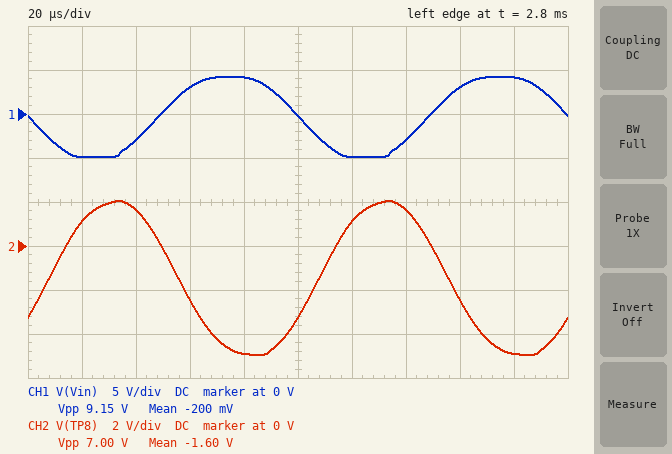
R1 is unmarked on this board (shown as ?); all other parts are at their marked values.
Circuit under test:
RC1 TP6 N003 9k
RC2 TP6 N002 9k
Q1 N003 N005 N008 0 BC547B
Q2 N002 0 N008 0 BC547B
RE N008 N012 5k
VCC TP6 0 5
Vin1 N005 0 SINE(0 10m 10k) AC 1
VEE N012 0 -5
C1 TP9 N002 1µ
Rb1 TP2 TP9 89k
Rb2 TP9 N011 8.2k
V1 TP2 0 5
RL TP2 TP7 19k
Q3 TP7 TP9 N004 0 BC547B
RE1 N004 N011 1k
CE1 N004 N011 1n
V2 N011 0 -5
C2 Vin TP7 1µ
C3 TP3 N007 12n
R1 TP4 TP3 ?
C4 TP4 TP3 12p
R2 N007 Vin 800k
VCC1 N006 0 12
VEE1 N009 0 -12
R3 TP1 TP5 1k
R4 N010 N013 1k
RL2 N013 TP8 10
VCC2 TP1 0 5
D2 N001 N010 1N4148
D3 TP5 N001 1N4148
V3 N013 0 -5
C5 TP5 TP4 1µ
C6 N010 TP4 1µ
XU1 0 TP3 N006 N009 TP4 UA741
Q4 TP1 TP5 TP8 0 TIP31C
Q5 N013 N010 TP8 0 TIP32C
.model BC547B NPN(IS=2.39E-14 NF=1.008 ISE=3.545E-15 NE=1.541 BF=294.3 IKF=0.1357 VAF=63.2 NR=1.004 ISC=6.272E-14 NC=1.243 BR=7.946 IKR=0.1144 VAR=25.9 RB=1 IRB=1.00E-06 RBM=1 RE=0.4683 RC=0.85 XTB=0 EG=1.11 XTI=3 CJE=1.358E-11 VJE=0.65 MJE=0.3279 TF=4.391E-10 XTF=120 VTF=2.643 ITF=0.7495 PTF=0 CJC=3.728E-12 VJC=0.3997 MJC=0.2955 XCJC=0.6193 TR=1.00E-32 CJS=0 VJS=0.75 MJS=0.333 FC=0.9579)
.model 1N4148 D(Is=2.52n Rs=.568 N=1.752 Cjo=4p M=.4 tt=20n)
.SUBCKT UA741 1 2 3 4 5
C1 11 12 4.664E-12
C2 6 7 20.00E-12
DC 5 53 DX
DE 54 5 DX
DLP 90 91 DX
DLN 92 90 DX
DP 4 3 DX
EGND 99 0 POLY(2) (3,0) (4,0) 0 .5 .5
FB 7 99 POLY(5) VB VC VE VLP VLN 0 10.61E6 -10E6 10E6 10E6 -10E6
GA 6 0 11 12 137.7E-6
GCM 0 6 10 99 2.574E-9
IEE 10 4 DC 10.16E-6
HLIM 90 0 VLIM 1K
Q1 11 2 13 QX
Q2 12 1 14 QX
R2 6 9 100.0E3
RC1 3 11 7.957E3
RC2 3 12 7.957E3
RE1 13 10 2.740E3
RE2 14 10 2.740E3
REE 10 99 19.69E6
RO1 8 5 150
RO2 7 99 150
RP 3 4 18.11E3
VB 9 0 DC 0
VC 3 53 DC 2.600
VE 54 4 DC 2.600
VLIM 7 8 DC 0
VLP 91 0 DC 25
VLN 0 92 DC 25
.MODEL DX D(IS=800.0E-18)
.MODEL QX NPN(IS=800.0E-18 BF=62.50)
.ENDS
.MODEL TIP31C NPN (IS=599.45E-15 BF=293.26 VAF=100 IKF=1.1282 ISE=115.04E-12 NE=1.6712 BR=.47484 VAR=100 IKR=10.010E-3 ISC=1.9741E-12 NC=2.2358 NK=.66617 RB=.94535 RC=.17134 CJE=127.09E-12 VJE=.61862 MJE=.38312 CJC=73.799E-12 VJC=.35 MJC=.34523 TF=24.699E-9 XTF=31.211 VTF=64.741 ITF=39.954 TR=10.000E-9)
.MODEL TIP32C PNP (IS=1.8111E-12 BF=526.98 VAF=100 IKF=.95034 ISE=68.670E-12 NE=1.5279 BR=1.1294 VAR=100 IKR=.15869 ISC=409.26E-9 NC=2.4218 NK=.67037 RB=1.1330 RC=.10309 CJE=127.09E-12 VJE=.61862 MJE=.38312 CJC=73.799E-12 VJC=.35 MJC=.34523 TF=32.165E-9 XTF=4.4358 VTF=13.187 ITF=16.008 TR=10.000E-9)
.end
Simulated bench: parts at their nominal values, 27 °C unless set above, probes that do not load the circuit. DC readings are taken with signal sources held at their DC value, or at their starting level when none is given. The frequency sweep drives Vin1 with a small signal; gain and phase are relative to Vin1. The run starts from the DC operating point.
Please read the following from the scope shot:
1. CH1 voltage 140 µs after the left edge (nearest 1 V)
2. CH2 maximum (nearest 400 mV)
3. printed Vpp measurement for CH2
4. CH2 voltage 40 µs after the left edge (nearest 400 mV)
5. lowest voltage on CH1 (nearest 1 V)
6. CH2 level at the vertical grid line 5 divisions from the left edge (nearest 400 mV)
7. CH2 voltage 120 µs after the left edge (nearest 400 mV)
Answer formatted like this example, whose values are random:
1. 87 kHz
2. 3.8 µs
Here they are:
1. -3 V
2. 2.0 V
3. 7.00 V
4. 1.6 V
5. -5 V
6. -3.2 V
7. 1.2 V
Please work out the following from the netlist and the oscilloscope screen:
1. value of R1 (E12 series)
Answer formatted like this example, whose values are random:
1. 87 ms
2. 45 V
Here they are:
1. 680 kΩ
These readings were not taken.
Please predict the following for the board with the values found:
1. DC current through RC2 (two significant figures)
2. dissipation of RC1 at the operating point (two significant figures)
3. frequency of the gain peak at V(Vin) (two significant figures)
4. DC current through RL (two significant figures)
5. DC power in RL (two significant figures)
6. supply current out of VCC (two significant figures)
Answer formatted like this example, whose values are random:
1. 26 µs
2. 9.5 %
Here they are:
1. 440 µA
2. 1.7 mW
3. 420 kHz
4. 240 µA
5. 1.1 mW
6. 870 µA
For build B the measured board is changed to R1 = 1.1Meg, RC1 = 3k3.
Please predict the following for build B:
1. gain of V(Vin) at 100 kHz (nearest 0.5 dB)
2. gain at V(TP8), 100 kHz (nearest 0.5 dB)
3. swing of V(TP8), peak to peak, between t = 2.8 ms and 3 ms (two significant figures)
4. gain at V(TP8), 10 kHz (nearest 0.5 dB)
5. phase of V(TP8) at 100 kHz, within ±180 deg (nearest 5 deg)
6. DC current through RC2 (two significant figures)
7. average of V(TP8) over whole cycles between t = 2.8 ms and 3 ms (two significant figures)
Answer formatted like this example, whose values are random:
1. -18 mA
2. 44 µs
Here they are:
1. 56.5 dB
2. 40.5 dB
3. 9.0 V
4. 55.0 dB
5. -70 deg
6. 430 µA
7. -1.0 V
